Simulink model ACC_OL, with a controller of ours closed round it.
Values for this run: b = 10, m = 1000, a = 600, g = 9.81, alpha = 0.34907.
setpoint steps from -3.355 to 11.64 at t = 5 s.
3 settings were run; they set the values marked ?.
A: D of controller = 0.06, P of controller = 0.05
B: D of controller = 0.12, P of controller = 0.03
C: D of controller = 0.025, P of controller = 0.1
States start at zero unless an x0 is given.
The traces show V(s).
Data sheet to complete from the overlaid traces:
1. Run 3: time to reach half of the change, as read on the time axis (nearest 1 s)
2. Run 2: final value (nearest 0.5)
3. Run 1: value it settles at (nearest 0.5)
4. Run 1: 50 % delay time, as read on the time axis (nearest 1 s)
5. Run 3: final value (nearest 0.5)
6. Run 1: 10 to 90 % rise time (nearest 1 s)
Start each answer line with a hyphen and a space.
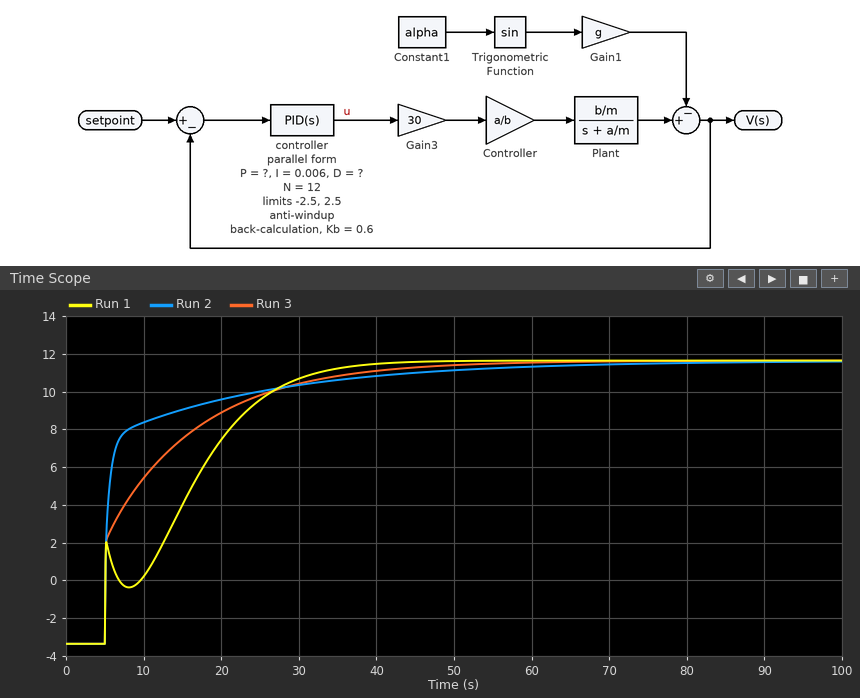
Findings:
- 8 s
- 11.5
- 11.5
- 15 s
- 11.5
- 22 s
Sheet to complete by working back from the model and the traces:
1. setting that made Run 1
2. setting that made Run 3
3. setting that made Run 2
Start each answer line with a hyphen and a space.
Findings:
- B
- A
- C
